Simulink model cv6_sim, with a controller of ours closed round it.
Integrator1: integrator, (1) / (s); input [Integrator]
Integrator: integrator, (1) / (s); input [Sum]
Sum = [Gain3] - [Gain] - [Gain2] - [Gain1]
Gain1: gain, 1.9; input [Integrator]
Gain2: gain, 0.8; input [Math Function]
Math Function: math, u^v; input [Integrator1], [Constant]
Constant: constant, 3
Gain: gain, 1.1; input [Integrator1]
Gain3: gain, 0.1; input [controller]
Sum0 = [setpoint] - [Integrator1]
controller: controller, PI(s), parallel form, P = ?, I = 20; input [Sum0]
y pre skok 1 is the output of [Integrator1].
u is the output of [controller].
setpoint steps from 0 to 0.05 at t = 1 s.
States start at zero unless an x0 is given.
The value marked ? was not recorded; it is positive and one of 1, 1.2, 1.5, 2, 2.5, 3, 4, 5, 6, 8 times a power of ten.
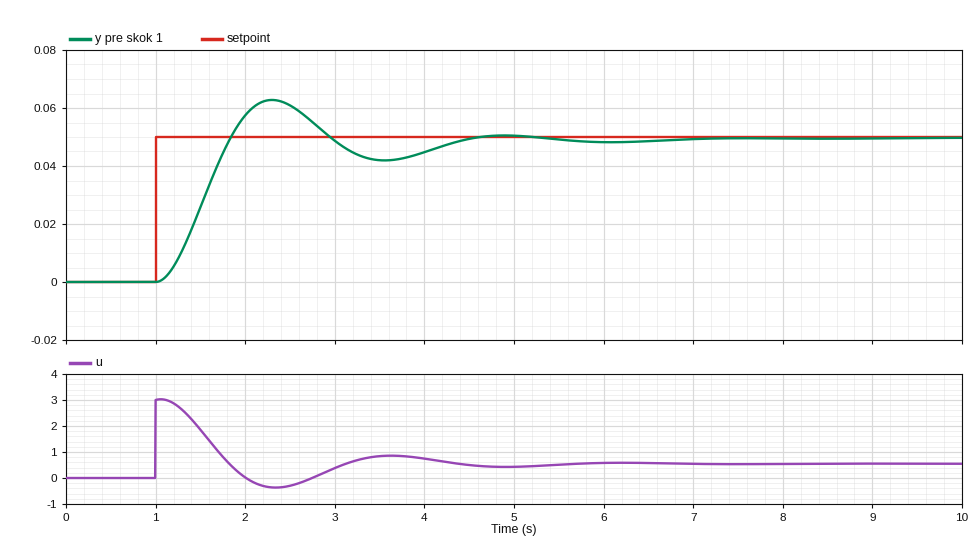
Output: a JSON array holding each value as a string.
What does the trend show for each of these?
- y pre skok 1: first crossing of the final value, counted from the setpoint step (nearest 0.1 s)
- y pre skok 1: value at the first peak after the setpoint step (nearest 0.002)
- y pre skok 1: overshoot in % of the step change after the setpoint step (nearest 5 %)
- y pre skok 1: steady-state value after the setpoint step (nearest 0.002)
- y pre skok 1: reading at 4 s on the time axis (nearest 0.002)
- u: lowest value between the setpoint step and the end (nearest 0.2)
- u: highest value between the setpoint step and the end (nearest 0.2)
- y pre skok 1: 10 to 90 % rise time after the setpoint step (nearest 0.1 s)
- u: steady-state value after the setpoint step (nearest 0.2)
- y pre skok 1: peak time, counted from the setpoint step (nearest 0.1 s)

["0.8 s", "0.062", "25 %", "0.050", "0.044", "-0.4", "3.0", "0.6 s", "0.6", "1.3 s"]
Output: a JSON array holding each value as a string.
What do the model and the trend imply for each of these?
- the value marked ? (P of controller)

["60"]
